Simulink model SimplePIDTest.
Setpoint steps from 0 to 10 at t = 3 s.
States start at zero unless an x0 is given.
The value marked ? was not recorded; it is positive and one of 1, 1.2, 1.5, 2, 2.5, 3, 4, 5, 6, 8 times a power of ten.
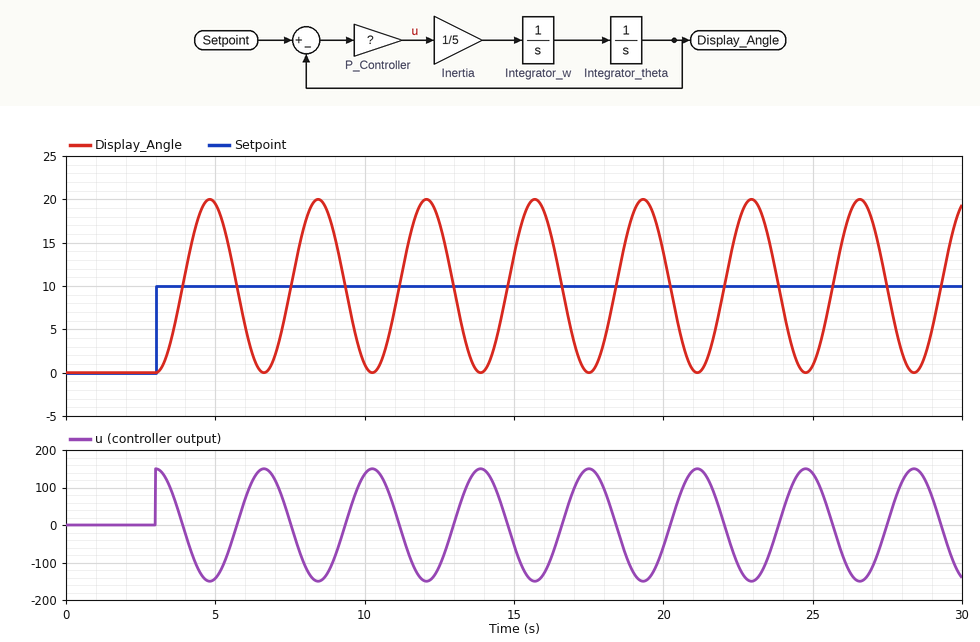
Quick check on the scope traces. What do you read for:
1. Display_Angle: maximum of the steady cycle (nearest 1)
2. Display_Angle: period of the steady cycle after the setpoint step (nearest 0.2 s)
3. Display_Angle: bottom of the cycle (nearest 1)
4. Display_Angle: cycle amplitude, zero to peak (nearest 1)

20
3.6 s
0
10
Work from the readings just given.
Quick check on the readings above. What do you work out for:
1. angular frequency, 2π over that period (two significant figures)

1.7 rad/s
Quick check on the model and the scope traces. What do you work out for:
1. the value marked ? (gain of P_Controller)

15
